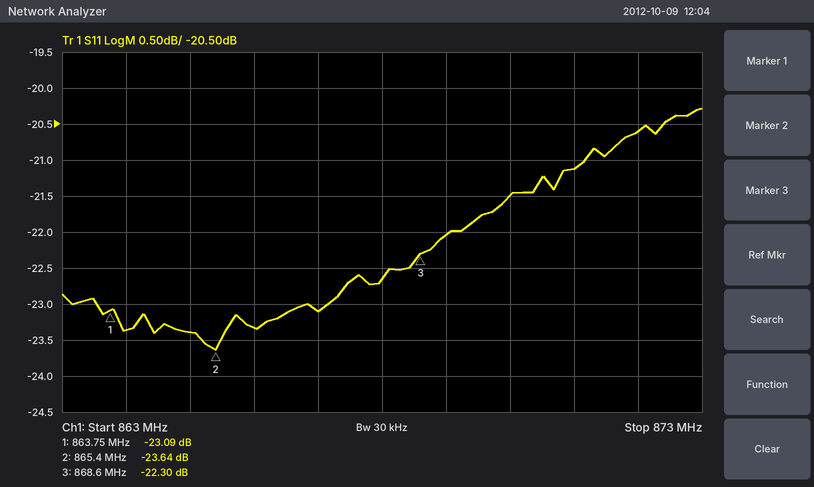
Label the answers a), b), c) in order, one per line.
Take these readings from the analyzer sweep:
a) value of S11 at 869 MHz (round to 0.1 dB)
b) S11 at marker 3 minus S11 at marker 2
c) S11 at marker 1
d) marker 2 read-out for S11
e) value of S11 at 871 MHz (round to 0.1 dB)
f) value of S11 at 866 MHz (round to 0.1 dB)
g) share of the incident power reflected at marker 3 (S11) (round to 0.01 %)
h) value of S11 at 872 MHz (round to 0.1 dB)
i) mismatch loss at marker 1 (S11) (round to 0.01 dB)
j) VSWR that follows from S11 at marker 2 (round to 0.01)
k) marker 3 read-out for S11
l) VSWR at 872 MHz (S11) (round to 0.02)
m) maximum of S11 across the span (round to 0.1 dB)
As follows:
a) -22.0 dB
b) 1.34 dB
c) -23.09 dB
d) -23.64 dB
e) -21.1 dB
f) -23.3 dB
g) 0.59 %
h) -20.6 dB
i) 0.02 dB
j) 1.14
k) -22.30 dB
l) 1.20
m) -20.3 dB
